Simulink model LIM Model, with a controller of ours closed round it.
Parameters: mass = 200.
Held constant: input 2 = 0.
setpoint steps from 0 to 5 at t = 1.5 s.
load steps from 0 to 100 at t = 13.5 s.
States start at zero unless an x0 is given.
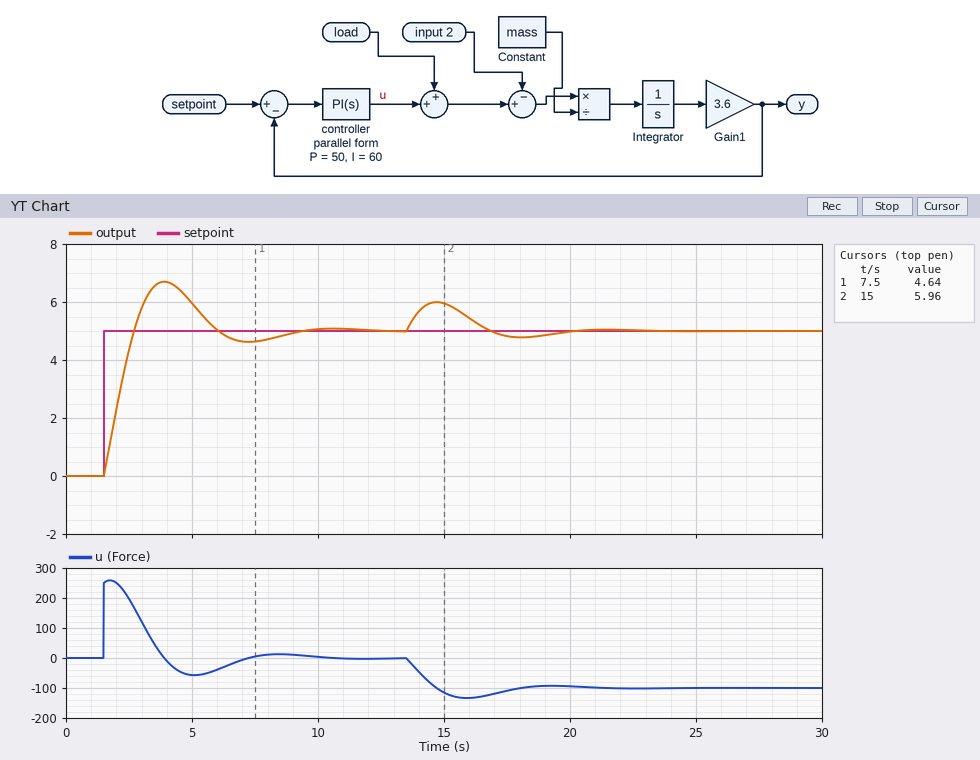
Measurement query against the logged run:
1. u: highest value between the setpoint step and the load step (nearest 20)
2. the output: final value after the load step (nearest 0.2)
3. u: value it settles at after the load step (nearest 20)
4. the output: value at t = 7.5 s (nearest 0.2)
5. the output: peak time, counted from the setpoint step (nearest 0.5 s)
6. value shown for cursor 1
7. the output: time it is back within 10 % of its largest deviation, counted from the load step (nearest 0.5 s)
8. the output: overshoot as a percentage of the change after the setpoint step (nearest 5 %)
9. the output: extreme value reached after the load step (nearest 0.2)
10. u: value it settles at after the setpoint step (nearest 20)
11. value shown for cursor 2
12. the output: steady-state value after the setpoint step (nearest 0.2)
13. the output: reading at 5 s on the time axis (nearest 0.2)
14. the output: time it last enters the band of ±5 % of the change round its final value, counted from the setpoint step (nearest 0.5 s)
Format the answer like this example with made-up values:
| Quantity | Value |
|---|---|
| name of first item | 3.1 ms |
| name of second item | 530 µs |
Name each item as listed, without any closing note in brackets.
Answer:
| Quantity | Value |
|---|---|
| u: highest value between the setpoint step and the load step | 260 |
| the output: final value after the load step | 5.0 |
| u: value it settles at after the load step | -100 |
| the output: value at t = 7.5 s | 4.6 |
| the output: peak time, counted from the setpoint step | 2.5 s |
| value shown for cursor 1 | 4.64 |
| the output: time it is back within 10 % of its largest deviation, counted from the load step | 6.0 s |
| the output: overshoot as a percentage of the change after the setpoint step | 35 % |
| the output: extreme value reached after the load step | 6.0 |
| u: value it settles at after the setpoint step | 0 |
| value shown for cursor 2 | 5.96 |
| the output: steady-state value after the setpoint step | 5.0 |
| the output: reading at 5 s on the time axis | 6.0 |
| the output: time it last enters the band of ±5 % of the change round its final value, counted from the setpoint step | 6.5 s |
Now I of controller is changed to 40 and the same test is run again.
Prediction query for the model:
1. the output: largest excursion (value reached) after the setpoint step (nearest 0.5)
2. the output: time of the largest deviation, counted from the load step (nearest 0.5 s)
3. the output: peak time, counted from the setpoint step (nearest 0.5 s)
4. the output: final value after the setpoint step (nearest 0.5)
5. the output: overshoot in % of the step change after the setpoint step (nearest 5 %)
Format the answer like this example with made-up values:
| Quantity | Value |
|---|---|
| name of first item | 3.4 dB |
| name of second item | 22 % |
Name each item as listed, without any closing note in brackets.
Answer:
| Quantity | Value |
|---|---|
| the output: largest excursion (value reached) after the setpoint step | 6.5 |
| the output: time of the largest deviation, counted from the load step | 1.5 s |
| the output: peak time, counted from the setpoint step | 3.0 s |
| the output: final value after the setpoint step | 5.0 |
| the output: overshoot in % of the step change after the setpoint step | 30 % |
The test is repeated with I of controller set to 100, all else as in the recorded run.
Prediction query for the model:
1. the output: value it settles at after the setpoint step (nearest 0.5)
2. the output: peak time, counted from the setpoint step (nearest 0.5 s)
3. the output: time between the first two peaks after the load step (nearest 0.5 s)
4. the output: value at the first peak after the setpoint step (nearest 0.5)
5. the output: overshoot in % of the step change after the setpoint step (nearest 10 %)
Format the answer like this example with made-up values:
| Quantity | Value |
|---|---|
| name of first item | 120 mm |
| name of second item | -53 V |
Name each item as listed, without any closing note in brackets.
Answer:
| Quantity | Value |
|---|---|
| the output: value it settles at after the setpoint step | 5.0 |
| the output: peak time, counted from the setpoint step | 2.0 s |
| the output: time between the first two peaks after the load step | 5.0 s |
| the output: value at the first peak after the setpoint step | 7.0 |
| the output: overshoot in % of the step change after the setpoint step | 40 % |
